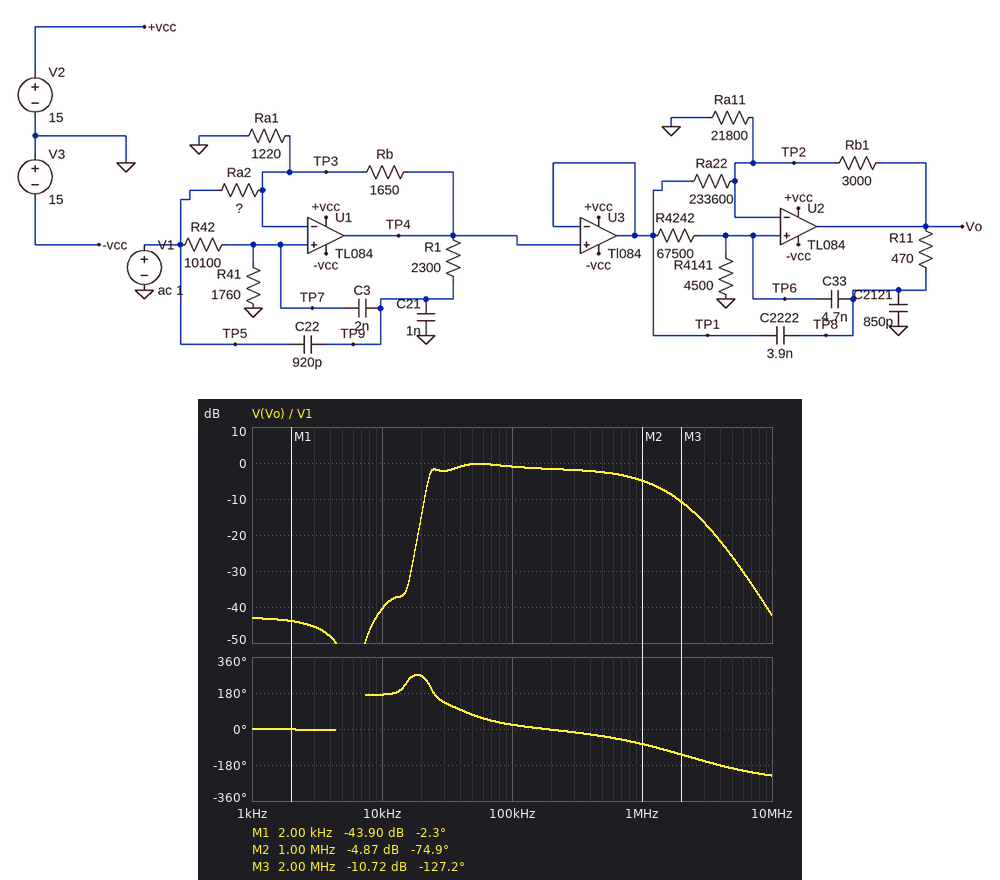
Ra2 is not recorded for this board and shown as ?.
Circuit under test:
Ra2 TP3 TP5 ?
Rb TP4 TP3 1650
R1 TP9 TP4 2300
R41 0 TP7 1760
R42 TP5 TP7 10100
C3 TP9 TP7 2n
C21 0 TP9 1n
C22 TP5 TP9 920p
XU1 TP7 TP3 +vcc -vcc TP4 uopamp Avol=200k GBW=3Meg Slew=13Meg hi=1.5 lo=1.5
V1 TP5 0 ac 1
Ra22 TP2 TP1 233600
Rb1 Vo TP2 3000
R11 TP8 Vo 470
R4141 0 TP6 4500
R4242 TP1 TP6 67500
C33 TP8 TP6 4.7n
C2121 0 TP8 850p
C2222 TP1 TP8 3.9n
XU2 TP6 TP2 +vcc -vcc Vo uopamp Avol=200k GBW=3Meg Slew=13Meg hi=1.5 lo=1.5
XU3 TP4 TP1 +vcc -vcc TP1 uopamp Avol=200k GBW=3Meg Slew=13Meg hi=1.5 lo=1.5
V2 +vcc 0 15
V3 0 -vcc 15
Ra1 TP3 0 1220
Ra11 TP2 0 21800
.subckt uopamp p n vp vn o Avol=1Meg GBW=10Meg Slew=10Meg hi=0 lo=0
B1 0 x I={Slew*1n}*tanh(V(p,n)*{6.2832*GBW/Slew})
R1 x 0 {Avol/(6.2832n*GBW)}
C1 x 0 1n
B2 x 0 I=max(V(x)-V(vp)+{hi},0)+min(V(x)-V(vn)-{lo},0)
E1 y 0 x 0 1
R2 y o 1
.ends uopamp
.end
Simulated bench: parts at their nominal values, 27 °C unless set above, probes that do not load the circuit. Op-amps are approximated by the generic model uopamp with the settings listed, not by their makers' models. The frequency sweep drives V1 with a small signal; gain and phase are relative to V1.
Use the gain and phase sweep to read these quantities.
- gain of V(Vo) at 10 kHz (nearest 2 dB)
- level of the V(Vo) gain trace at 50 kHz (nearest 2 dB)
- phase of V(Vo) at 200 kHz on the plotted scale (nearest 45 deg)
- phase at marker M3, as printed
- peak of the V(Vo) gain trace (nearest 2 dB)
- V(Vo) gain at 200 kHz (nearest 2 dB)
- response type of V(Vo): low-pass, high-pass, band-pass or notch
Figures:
-40 dB
0 dB
0 deg
-127.2 deg
0 dB
-2 dB
band-pass
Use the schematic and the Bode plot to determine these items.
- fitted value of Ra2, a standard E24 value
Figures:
6.2 kΩ
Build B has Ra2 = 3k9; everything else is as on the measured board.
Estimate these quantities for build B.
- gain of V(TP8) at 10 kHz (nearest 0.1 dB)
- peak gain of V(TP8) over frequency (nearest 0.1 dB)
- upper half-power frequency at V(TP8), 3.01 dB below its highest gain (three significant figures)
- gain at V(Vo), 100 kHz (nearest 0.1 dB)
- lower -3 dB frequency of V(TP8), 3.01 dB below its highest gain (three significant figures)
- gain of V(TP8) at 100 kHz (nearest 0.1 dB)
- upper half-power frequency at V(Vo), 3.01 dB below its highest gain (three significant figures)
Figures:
-35.0 dB
3.4 dB
48.5 kHz
-1.2 dB
22.2 kHz
-2.3 dB
53.2 kHz
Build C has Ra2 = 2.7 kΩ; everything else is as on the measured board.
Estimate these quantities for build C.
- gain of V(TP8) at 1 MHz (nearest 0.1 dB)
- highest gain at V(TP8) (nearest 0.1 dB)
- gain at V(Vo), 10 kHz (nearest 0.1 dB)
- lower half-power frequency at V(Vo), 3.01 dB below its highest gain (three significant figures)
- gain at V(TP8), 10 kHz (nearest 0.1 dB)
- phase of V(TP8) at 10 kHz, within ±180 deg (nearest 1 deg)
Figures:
-7.6 dB
9.3 dB
-28.1 dB
22.1 kHz
-25.7 dB
-26 deg
